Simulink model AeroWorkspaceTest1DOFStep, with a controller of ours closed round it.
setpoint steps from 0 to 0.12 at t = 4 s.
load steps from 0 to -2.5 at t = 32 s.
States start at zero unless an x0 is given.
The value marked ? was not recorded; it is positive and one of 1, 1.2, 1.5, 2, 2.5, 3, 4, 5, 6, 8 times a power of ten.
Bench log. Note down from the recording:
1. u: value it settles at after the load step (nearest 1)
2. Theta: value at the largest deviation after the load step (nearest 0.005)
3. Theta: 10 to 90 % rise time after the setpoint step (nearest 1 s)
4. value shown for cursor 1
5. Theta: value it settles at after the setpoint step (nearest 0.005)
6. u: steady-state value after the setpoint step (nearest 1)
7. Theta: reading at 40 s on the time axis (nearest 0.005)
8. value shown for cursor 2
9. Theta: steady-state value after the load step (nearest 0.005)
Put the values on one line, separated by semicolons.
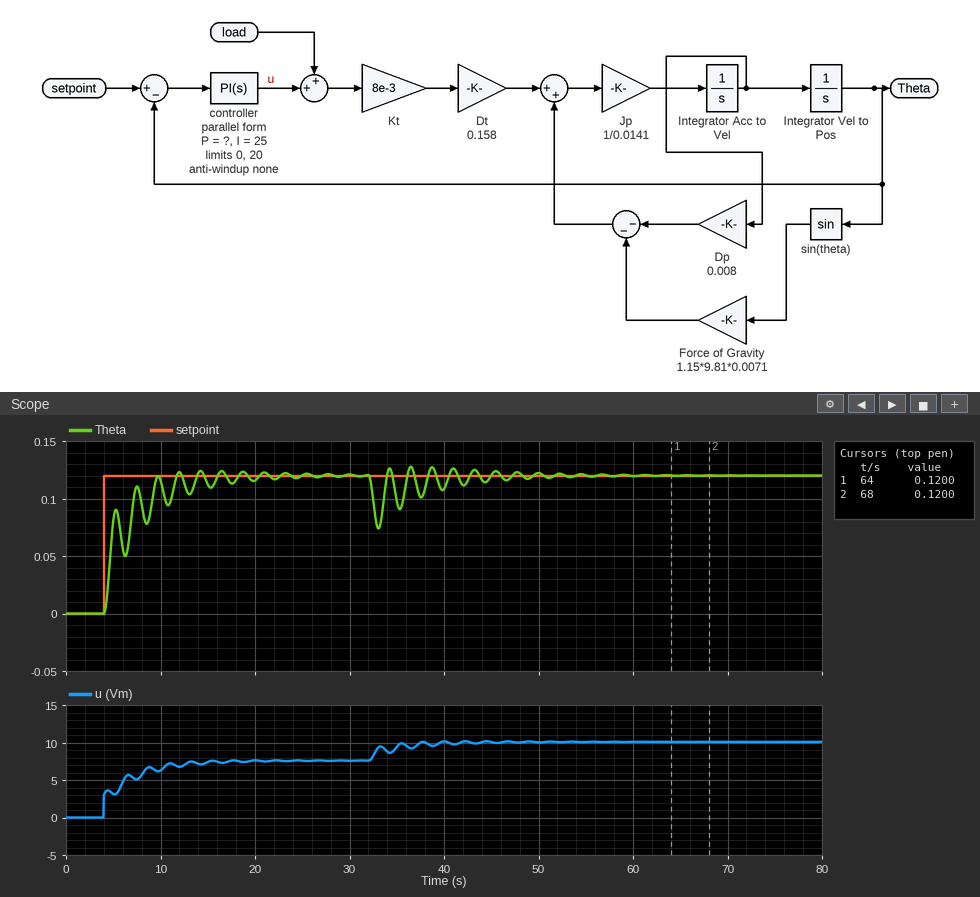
10; 0.075; 3 s; 0.1200; 0.120; 8; 0.110; 0.1200; 0.120
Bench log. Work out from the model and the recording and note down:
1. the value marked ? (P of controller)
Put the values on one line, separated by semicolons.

25
